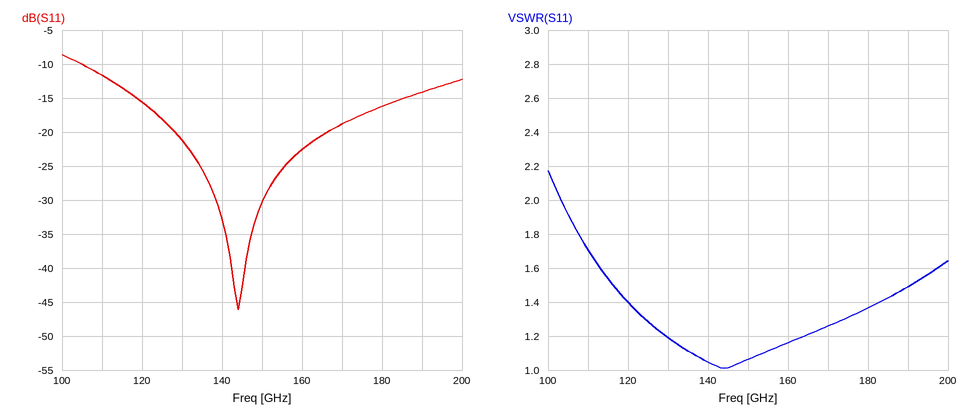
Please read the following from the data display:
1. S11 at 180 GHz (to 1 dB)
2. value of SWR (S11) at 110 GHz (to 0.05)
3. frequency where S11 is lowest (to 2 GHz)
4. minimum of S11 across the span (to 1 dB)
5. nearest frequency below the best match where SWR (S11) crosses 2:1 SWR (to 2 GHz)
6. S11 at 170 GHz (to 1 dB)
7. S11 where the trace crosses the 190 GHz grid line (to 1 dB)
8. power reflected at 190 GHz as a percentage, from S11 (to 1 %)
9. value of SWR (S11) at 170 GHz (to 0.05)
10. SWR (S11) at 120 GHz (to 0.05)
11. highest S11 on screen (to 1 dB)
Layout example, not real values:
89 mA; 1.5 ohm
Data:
-16 dB; 1.70; 144 GHz; -46 dB; 104 GHz; -19 dB; -14 dB; 4 %; 1.25; 1.40; -9 dB
